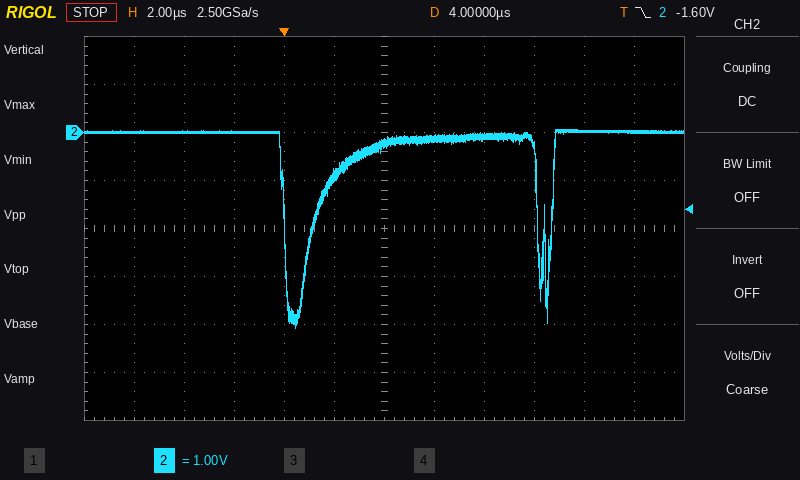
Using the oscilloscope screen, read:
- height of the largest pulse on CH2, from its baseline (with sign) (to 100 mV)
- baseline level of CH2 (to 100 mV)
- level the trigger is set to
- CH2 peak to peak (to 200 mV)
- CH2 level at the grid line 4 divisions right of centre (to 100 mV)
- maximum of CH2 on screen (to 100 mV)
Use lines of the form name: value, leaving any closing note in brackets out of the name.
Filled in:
height of the largest pulse on CH2, from its baseline (with sign): -4.1 V
baseline level of CH2: 0.0 V
level the trigger is set to: -1.60 V
CH2 peak to peak: 4.2 V
CH2 level at the grid line 4 divisions right of centre: 0.0 V
maximum of CH2 on screen: 100 mV
